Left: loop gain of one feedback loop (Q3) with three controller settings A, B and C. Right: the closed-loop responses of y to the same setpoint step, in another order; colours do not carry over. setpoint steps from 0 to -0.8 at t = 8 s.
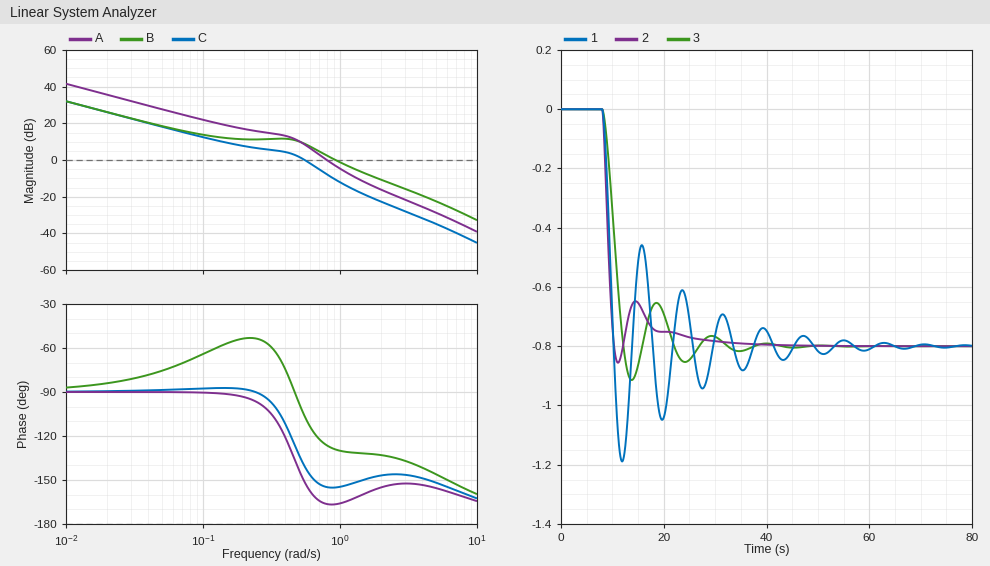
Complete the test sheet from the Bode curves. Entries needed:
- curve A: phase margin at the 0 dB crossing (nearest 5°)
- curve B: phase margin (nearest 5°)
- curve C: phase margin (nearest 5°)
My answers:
15°
50°
40°
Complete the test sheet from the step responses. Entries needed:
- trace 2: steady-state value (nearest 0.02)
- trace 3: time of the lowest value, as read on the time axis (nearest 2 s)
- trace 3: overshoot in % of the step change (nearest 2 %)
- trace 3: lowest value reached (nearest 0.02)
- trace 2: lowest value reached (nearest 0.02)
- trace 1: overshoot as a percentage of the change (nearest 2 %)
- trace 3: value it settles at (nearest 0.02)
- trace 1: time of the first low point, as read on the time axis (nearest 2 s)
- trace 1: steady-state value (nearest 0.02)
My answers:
-0.80
14 s
14 %
-0.92
-0.86
48 %
-0.80
12 s
-0.80
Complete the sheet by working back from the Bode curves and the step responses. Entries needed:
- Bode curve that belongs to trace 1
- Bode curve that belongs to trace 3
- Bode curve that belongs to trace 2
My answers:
A
C
B
